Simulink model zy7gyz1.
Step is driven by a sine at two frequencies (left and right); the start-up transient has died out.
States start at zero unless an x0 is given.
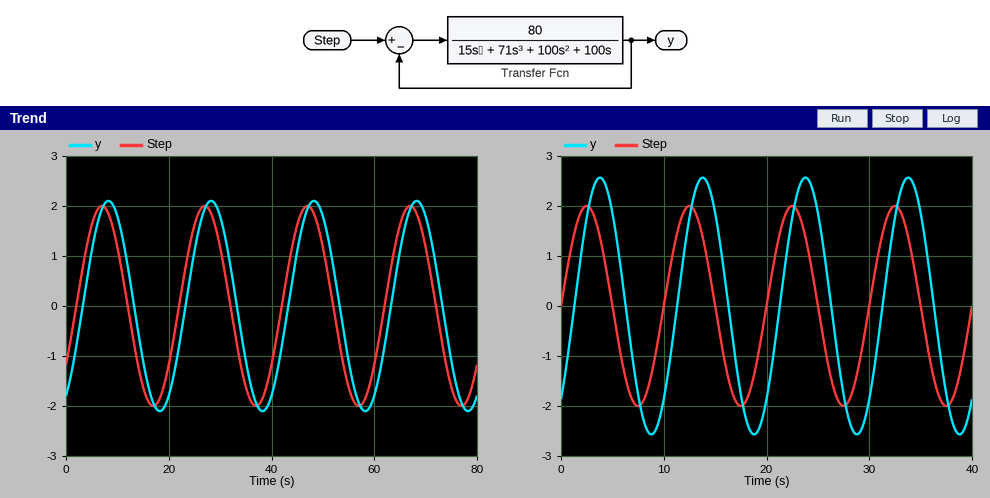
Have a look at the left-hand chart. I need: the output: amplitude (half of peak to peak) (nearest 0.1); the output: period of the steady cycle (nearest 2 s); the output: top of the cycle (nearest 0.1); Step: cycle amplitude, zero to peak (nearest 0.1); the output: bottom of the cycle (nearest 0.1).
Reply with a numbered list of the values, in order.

1. 2.1
2. 20 s
3. 2.1
4. 2.0
5. -2.1
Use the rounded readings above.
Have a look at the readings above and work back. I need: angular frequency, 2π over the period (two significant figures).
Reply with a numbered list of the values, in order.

1. 0.31 rad/s
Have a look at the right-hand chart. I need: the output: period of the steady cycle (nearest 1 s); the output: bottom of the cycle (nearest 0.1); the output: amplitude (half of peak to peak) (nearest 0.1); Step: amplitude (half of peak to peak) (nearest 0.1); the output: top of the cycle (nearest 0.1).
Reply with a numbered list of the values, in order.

1. 10 s
2. -2.6
3. 2.6
4. 2.0
5. 2.6
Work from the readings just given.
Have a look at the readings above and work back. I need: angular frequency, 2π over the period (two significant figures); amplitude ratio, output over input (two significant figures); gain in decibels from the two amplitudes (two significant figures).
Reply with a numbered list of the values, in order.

1. 0.63 rad/s
2. 1.3
3. 2.3 dB
